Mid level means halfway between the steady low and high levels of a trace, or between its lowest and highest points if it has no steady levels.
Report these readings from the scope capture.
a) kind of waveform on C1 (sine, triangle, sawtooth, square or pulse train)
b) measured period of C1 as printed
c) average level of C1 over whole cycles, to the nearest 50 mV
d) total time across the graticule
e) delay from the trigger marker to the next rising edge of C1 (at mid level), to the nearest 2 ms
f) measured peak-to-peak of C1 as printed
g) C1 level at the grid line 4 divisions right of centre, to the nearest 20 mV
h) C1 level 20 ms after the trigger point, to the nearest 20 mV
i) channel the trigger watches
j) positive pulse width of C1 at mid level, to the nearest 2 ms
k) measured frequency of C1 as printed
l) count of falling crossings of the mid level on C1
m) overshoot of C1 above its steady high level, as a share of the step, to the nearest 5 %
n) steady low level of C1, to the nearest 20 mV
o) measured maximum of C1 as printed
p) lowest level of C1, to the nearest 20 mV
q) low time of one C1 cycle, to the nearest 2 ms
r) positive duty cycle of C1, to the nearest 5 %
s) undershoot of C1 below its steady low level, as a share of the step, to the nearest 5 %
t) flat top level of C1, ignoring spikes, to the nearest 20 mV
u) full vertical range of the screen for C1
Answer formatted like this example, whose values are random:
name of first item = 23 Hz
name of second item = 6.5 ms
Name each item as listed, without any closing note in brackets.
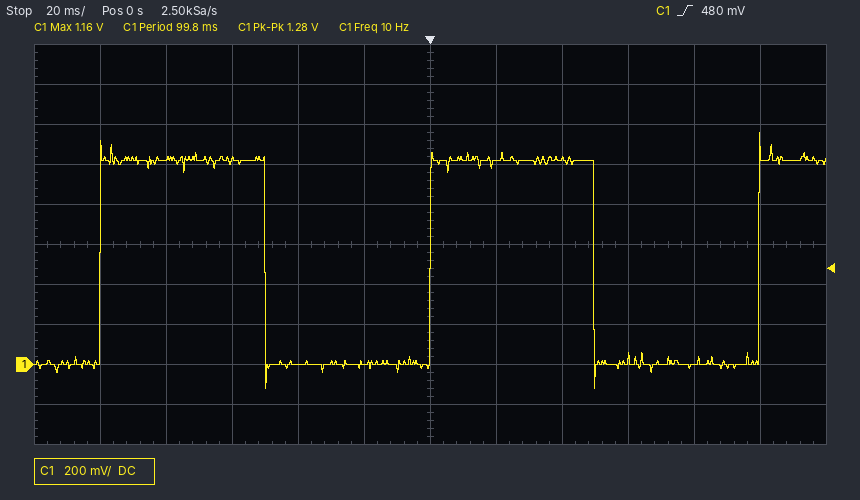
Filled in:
kind of waveform on C1 = square
measured period of C1 as printed = 99.8 ms
average level of C1 over whole cycles, to the nearest 50 mV = 500 mV
total time across the graticule = 240 ms
delay from the trigger marker to the next rising edge of C1 (at mid level), to the nearest 2 ms = 100 ms
measured peak-to-peak of C1 as printed = 1.28 V
C1 level at the grid line 4 divisions right of centre, to the nearest 20 mV = 0 mV
C1 level 20 ms after the trigger point, to the nearest 20 mV = 1.02 V
channel the trigger watches = C1
positive pulse width of C1 at mid level, to the nearest 2 ms = 50 ms
measured frequency of C1 as printed = 10 Hz
count of falling crossings of the mid level on C1 = 2
overshoot of C1 above its steady high level, as a share of the step, to the nearest 5 % = 15 %
steady low level of C1, to the nearest 20 mV = 0 mV
measured maximum of C1 as printed = 1.16 V
lowest level of C1, to the nearest 20 mV = -120 mV
low time of one C1 cycle, to the nearest 2 ms = 50 ms
positive duty cycle of C1, to the nearest 5 % = 50 %
undershoot of C1 below its steady low level, as a share of the step, to the nearest 5 % = 10 %
flat top level of C1, ignoring spikes, to the nearest 20 mV = 1.02 V
full vertical range of the screen for C1 = 2 V
